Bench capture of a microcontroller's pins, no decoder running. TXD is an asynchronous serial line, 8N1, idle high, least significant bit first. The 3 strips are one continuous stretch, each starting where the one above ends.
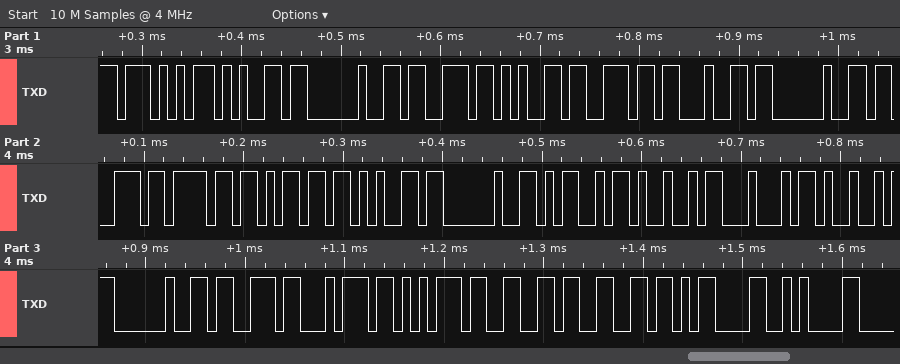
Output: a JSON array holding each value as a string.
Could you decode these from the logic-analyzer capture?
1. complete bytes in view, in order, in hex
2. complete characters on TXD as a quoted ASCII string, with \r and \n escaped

["57 65 20 73 65 6E 64 20 73 6F 6D 65 20 4D 49 44 49 20 73 74 75 66 66 0D 0A", "\"We send some MIDI stuff\\r\\n\""]
